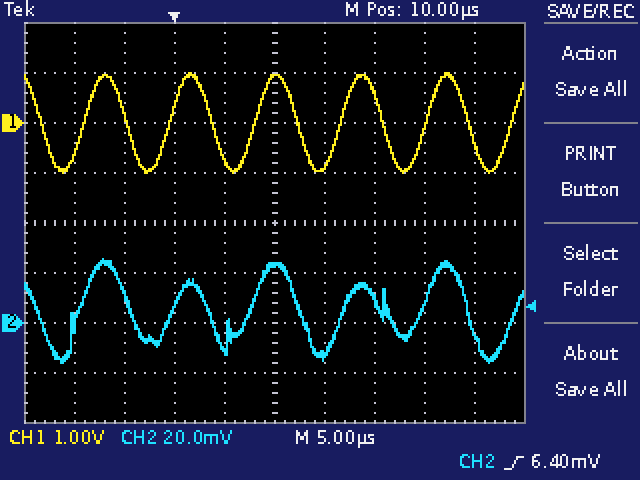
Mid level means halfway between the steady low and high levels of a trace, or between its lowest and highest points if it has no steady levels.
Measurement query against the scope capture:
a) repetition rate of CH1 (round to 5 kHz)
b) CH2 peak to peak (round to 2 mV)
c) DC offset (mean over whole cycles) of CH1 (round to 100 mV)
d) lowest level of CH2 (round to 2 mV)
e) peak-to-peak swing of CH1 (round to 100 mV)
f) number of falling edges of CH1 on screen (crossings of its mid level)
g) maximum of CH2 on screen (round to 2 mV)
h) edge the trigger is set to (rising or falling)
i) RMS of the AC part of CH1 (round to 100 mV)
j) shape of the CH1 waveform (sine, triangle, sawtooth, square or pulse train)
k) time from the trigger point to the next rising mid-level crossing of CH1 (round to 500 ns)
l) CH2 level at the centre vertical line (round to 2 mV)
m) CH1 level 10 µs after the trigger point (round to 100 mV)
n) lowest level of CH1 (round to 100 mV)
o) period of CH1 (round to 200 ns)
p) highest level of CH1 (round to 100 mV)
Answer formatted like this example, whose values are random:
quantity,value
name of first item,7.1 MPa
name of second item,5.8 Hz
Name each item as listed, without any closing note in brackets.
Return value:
quantity,value
repetition rate of CH1,115 kHz
CH2 peak to peak,42 mV
DC offset (mean over whole cycles) of CH1,0.0 V
lowest level of CH2,-16 mV
peak-to-peak swing of CH1,2.0 V
number of falling edges of CH1 on screen,6
maximum of CH2 on screen,26 mV
edge the trigger is set to,rising
RMS of the AC part of CH1,700 mV
shape of the CH1 waveform,sine
time from the trigger point to the next rising mid-level crossing of CH1,8.0 µs
CH2 level at the centre vertical line,24 mV
CH1 level 10 µs after the trigger point,900 mV
lowest level of CH1,-1.0 V
period of CH1,8.6 µs
highest level of CH1,1.0 V
